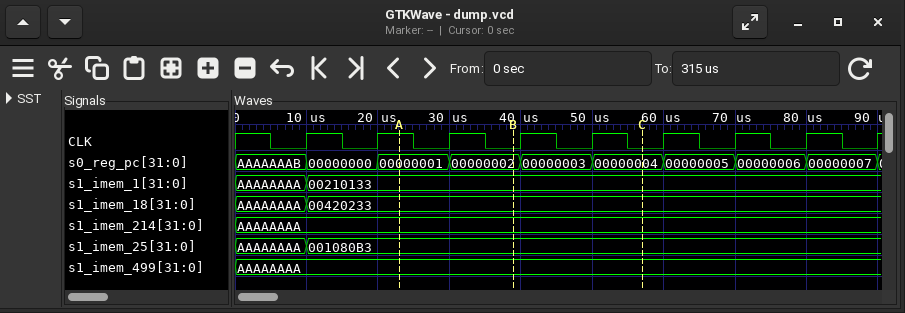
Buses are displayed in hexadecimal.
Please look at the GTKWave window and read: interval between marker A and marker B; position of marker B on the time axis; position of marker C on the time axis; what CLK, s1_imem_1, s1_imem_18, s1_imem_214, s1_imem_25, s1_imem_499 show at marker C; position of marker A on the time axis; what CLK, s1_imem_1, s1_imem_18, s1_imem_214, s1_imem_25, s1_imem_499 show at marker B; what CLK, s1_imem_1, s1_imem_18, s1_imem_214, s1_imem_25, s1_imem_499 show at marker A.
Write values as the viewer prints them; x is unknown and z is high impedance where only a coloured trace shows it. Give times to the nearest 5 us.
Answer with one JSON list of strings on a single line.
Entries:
["15 us", "40 us", "55 us", "CLK=0, s1_imem_1=00210133, s1_imem_18=00420233, s1_imem_214=AAAAAAAA, s1_imem_25=001080B3, s1_imem_499=AAAAAAAA", "25 us", "CLK=0, s1_imem_1=00210133, s1_imem_18=00420233, s1_imem_214=AAAAAAAA, s1_imem_25=001080B3, s1_imem_499=AAAAAAAA", "CLK=1, s1_imem_1=00210133, s1_imem_18=00420233, s1_imem_214=AAAAAAAA, s1_imem_25=001080B3, s1_imem_499=AAAAAAAA"]
